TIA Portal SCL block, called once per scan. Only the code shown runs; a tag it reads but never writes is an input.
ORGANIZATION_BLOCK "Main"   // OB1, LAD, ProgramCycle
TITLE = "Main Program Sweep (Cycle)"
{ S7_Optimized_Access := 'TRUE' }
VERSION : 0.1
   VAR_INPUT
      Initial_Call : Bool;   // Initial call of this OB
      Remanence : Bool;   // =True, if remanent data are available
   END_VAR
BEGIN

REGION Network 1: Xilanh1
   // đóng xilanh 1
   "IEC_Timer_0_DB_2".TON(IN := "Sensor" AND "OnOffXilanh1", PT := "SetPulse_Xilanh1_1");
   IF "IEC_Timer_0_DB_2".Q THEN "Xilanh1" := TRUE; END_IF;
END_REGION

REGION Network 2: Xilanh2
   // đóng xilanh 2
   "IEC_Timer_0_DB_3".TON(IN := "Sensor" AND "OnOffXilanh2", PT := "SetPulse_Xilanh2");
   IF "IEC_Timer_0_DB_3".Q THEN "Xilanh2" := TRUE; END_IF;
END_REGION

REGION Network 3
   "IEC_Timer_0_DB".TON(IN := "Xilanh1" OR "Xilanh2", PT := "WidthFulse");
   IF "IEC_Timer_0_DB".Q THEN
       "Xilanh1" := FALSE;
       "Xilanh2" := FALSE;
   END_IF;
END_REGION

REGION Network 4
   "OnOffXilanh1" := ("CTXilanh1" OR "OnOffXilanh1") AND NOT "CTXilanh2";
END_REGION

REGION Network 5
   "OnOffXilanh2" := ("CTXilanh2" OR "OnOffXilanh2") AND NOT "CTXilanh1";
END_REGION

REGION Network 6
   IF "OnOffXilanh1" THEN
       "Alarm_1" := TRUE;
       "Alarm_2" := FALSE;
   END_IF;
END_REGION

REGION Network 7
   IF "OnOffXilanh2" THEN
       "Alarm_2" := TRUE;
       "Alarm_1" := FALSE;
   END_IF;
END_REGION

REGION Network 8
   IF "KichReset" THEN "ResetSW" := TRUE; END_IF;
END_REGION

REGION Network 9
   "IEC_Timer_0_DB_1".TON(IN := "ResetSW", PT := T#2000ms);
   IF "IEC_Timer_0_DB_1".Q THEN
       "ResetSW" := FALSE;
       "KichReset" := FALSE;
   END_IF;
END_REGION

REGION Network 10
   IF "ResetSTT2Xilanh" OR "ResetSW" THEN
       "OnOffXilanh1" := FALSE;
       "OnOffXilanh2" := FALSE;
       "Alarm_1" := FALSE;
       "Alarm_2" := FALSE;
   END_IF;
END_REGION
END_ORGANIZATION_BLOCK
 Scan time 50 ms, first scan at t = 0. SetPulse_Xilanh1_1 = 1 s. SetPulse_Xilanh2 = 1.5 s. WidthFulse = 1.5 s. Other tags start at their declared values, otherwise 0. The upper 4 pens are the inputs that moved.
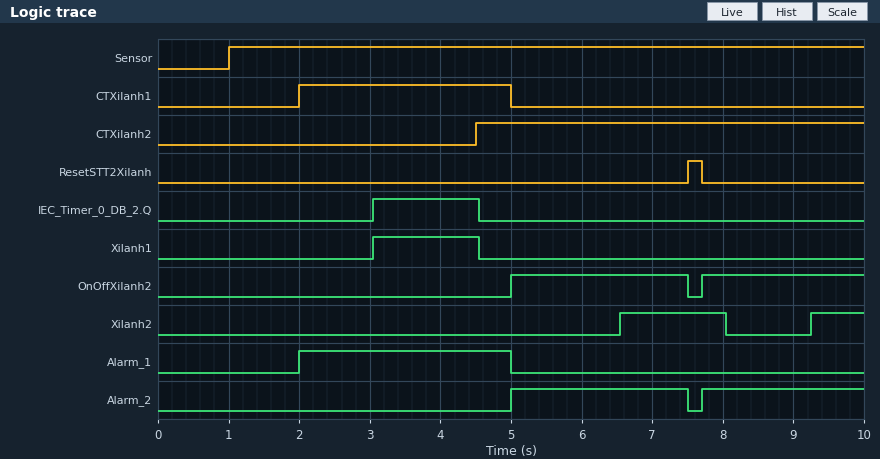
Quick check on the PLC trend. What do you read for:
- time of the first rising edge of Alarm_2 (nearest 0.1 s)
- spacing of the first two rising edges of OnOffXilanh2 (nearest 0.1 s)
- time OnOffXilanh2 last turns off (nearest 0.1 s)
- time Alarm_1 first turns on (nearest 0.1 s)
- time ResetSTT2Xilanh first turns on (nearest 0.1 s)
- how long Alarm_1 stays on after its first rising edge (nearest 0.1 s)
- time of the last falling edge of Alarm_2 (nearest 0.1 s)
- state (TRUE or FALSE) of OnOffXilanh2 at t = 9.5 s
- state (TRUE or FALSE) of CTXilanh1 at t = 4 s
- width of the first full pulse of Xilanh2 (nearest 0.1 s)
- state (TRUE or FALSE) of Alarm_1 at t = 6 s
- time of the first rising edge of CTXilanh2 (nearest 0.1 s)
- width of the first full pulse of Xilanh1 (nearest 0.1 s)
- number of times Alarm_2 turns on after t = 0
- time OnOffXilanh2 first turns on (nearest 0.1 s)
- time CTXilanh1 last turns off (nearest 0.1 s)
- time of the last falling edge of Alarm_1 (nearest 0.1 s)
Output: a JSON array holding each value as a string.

["5.0 s", "2.7 s", "7.5 s", "2.0 s", "7.5 s", "3.0 s", "7.5 s", "TRUE", "TRUE", "1.5 s", "FALSE", "4.5 s", "1.5 s", "2", "5.0 s", "5.0 s", "5.0 s"]
